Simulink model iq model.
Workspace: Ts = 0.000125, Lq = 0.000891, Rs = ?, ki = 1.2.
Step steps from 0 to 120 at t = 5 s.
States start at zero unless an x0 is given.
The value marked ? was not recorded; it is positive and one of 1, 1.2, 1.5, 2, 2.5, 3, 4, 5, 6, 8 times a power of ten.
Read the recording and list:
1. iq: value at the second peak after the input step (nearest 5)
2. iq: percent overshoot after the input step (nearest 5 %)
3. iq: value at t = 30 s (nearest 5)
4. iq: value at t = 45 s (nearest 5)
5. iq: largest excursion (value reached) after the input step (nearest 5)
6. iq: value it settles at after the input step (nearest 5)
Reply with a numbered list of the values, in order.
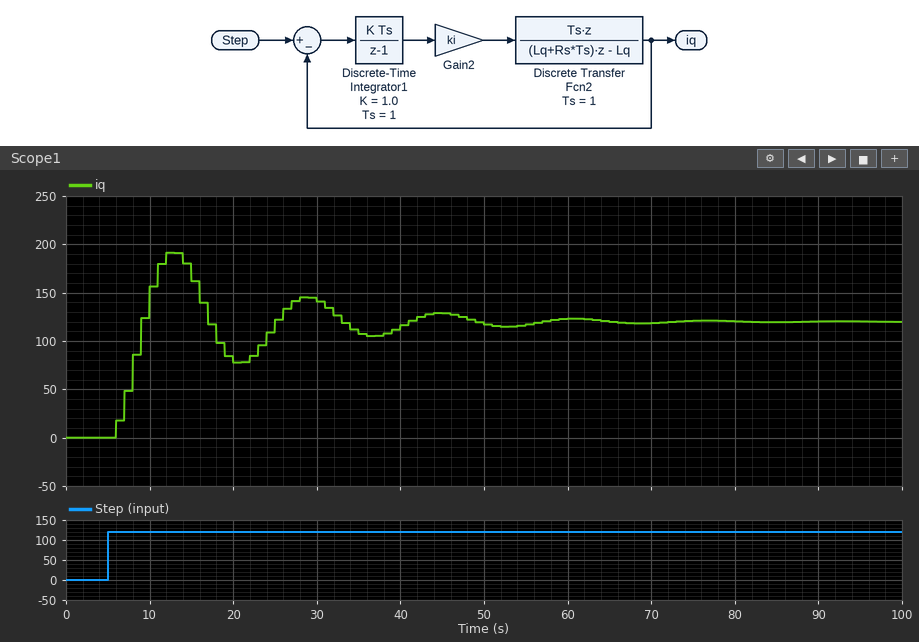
1. 145
2. 60 %
3. 140
4. 130
5. 190
6. 120
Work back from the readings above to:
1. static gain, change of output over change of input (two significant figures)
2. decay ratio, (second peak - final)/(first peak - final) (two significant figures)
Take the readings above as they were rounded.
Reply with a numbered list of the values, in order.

1. 1.0
2. 0.36
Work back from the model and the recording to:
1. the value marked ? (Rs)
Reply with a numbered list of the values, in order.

1. 1
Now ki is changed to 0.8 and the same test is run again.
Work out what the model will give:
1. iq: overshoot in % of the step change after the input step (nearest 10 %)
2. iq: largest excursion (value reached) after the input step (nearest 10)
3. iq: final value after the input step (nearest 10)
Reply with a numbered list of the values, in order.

1. 50 %
2. 180
3. 120
